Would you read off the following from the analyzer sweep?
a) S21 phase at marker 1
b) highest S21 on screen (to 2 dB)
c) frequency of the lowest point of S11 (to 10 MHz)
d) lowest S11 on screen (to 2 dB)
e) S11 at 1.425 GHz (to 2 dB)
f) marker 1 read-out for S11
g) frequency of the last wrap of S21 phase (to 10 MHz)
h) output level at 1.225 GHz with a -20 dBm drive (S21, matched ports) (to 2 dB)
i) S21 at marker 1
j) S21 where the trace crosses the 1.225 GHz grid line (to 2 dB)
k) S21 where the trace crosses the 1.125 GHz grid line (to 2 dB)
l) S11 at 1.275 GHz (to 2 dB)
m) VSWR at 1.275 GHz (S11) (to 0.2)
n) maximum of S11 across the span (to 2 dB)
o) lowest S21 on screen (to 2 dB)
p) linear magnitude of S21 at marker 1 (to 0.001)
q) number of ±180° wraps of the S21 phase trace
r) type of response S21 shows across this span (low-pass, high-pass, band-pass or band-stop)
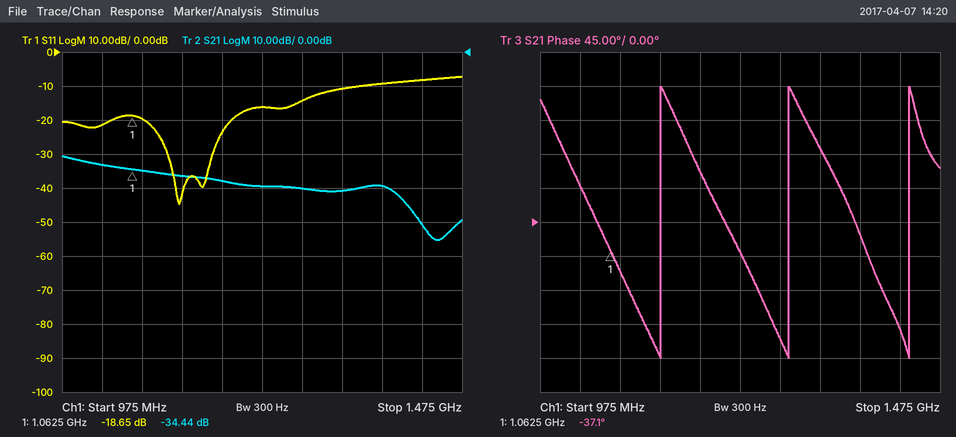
-37.1°
-30 dB
1.12 GHz
-44 dB
-8 dB
-18.65 dB
1.44 GHz
-60 dBm
-34.44 dB
-40 dB
-36 dB
-14 dB
1.4
-8 dB
-56 dB
0.019
3
low-pass
